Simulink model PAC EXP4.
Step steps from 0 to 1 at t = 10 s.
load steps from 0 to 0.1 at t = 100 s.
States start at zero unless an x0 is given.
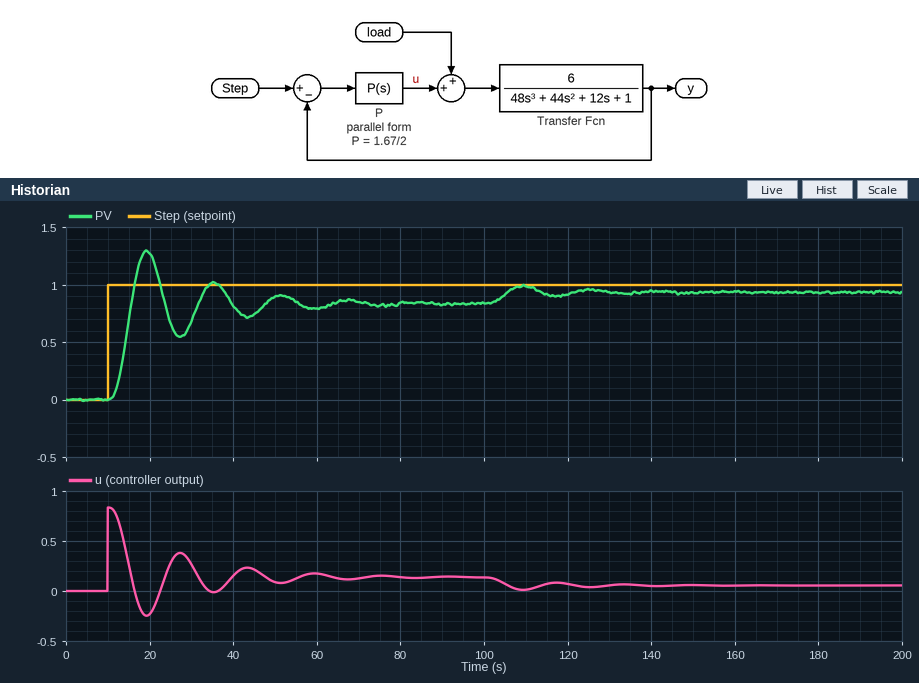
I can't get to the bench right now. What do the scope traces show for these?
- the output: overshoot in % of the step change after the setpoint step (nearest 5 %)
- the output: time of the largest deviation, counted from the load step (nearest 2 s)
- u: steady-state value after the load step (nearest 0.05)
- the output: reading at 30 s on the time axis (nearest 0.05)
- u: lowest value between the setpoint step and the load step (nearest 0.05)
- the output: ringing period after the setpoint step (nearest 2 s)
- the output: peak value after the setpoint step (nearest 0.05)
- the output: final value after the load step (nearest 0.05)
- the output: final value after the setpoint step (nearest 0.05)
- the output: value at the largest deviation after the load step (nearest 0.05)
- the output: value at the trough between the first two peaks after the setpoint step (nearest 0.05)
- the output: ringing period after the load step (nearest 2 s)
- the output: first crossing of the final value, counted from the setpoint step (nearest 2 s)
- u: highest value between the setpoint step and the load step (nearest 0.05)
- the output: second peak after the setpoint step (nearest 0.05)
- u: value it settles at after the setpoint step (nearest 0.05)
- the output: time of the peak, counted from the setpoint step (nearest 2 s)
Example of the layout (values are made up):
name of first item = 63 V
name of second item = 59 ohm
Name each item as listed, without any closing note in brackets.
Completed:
the output: overshoot in % of the step change after the setpoint step = 55 %
the output: time of the largest deviation, counted from the load step = 10 s
u: steady-state value after the load step = 0.05
the output: reading at 30 s on the time axis = 0.70
u: lowest value between the setpoint step and the load step = -0.25
the output: ringing period after the setpoint step = 16 s
the output: peak value after the setpoint step = 1.30
the output: final value after the load step = 0.95
the output: final value after the setpoint step = 0.85
the output: value at the largest deviation after the load step = 1.00
the output: value at the trough between the first two peaks after the setpoint step = 0.55
the output: ringing period after the load step = 16 s
the output: first crossing of the final value, counted from the setpoint step = 6 s
u: highest value between the setpoint step and the load step = 0.85
the output: second peak after the setpoint step = 1.00
u: value it settles at after the setpoint step = 0.15
the output: time of the peak, counted from the setpoint step = 10 s
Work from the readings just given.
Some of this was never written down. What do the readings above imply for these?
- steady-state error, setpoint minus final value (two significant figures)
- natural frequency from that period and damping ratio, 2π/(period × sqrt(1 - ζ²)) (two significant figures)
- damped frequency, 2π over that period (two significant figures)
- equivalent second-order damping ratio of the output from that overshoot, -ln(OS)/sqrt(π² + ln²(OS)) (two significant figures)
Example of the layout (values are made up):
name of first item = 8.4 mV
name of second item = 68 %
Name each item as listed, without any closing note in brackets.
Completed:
steady-state error, setpoint minus final value = 0.15
natural frequency from that period and damping ratio, 2π/(period × sqrt(1 - ζ²)) = 0.40 rad/s
damped frequency, 2π over that period = 0.39 rad/s
equivalent second-order damping ratio of the output from that overshoot, -ln(OS)/sqrt(π² + ln²(OS)) = 0.19
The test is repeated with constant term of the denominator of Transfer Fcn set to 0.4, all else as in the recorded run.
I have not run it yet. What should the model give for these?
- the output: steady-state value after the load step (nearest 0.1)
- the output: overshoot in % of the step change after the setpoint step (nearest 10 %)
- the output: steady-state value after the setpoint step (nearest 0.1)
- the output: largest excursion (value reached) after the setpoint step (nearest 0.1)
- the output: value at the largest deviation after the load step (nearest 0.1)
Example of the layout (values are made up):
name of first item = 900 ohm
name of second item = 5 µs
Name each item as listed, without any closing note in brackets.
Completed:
the output: steady-state value after the load step = 1.0
the output: overshoot in % of the step change after the setpoint step = 50 %
the output: steady-state value after the setpoint step = 0.9
the output: largest excursion (value reached) after the setpoint step = 1.4
the output: value at the largest deviation after the load step = 1.1
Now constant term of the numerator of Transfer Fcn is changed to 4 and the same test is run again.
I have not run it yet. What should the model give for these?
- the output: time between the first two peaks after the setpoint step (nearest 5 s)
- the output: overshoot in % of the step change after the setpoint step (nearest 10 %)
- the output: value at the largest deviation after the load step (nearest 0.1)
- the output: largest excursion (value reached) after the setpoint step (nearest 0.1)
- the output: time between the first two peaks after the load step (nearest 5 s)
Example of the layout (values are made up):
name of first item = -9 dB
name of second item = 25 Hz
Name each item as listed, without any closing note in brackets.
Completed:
the output: time between the first two peaks after the setpoint step = 20 s
the output: overshoot in % of the step change after the setpoint step = 40 %
the output: value at the largest deviation after the load step = 0.9
the output: largest excursion (value reached) after the setpoint step = 1.1
the output: time between the first two peaks after the load step = 20 s
